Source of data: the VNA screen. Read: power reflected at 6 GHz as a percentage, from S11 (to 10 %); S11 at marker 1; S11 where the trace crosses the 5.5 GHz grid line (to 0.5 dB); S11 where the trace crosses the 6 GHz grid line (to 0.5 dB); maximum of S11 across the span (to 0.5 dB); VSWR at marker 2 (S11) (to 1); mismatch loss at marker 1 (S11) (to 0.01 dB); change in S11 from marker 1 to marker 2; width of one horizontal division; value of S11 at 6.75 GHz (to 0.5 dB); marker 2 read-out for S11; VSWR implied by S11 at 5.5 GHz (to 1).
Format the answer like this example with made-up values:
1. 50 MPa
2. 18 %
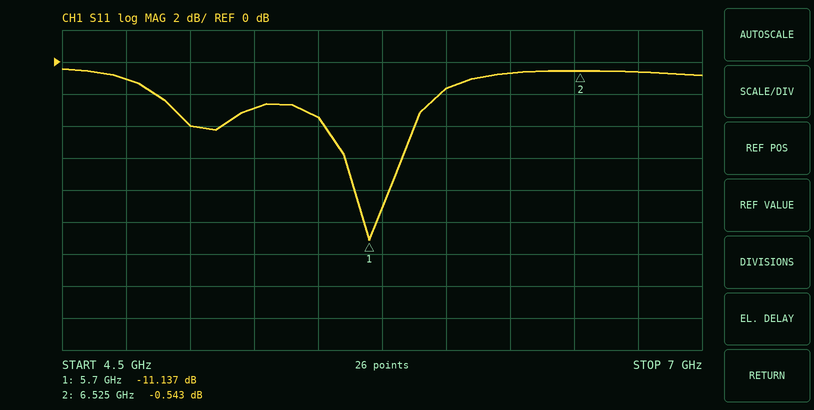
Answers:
1. 70 %
2. -11.137 dB
3. -3.5 dB
4. -1.5 dB
5. -0.5 dB
6. 32
7. 0.35 dB
8. 10.594 dB
9. 250 MHz
10. -0.5 dB
11. -0.543 dB
12. 5
